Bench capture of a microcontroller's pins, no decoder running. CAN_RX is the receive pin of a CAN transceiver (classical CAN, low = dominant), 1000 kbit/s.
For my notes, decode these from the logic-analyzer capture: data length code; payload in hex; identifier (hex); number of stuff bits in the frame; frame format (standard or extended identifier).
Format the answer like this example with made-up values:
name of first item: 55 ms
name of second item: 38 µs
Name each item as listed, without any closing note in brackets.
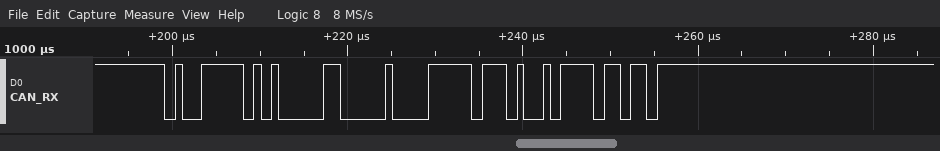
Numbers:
data length code: 2
payload in hex: 00 FF
identifier: 0x4FD
number of stuff bits in the frame: 4
frame format: standard
